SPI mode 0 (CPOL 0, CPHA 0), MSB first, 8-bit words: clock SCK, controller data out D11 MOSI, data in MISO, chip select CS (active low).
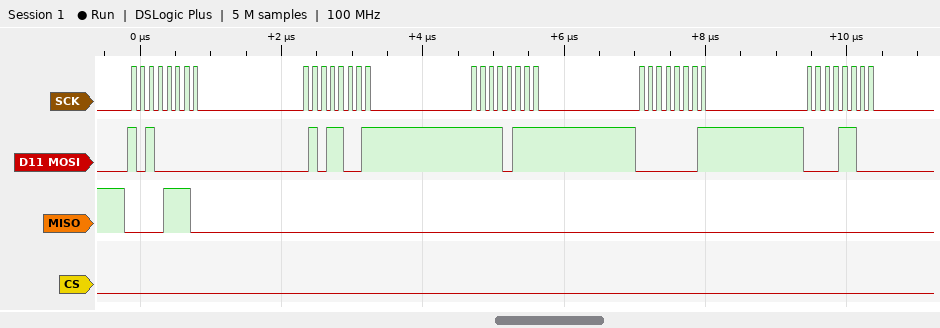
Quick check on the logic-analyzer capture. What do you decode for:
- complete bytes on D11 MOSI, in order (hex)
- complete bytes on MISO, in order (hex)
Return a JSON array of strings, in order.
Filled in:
["A0 59 F7 01 0C", "0E 00 00 00 00"]
